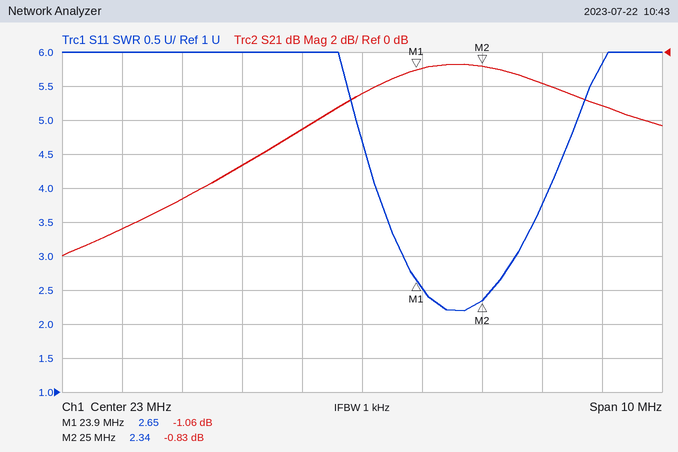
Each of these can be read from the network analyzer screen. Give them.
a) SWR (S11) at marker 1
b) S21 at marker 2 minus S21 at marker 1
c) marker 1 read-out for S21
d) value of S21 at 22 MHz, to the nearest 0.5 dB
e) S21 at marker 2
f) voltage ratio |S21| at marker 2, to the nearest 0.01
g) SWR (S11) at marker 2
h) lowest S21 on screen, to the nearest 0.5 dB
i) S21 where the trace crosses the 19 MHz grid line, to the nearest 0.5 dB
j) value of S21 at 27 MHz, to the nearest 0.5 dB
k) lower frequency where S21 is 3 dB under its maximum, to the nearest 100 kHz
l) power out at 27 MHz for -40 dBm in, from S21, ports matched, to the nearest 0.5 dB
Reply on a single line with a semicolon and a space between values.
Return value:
2.65; 0.23 dB; -1.06 dB; -4.5 dB; -0.83 dB; 0.91; 2.34; -12.0 dB; -10.5 dB; -3.0 dB; 22.4 MHz; -43.0 dBm
